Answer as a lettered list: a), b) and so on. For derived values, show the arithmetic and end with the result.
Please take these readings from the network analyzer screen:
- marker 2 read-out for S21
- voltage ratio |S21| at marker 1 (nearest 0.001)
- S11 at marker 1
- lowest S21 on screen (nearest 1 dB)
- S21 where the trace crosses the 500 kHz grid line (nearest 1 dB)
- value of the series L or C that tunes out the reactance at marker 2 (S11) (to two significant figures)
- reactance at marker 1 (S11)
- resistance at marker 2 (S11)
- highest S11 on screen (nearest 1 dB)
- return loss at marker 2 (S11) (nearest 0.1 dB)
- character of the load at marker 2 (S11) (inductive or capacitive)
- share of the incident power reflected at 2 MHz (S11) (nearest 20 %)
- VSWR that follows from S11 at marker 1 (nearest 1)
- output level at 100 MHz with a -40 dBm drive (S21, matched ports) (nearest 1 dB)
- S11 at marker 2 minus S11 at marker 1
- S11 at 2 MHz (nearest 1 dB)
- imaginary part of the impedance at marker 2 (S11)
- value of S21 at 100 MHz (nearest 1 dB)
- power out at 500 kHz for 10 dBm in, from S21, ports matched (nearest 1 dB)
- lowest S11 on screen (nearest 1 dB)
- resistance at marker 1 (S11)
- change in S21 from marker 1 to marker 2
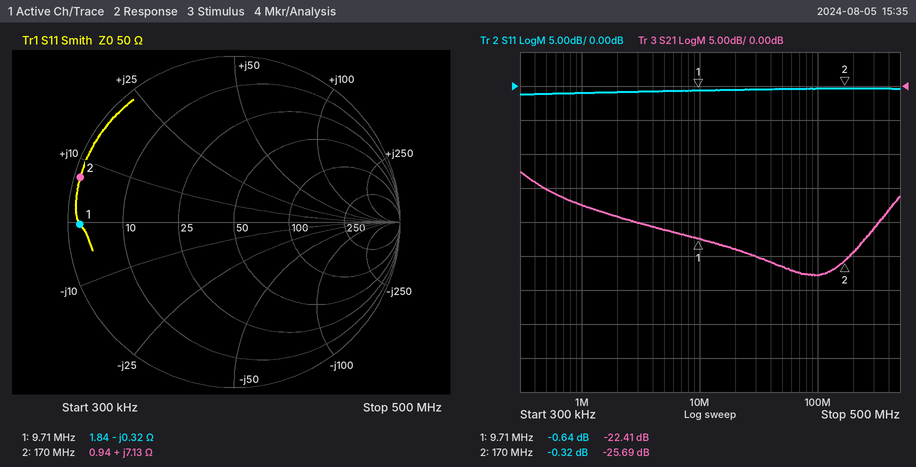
a) -25.69 dB
b) 10^(-22.41/20) ≈ 0.076
c) -0.64 dB
d) -28 dB
e) -15 dB
f) C = 1/(2π × 170 MHz × 7.13 Ω) ≈ 131 pF, so 130 pF to two significant figures
g) -0.32 Ω
h) 0.94 Ω
i) 0 dB
j) 0.3 dB
k) inductive
l) 10^(-1/10) ≈ 79.4 %, so 80 % to the nearest 20 %
m) (1 + 0.9290)/(1 − 0.9290) ≈ 27
n) -40 dBm + (-28 dB) = -68 dBm
o) -0.32 − (-0.64) = 0.32 dB
p) -1 dB
q) +7.13 Ω
r) -28 dB
s) 10 dBm + (-15 dB) = -5 dBm
t) -1 dB
u) 1.84 Ω
v) -25.69 − (-22.41) = -3.28 dB
